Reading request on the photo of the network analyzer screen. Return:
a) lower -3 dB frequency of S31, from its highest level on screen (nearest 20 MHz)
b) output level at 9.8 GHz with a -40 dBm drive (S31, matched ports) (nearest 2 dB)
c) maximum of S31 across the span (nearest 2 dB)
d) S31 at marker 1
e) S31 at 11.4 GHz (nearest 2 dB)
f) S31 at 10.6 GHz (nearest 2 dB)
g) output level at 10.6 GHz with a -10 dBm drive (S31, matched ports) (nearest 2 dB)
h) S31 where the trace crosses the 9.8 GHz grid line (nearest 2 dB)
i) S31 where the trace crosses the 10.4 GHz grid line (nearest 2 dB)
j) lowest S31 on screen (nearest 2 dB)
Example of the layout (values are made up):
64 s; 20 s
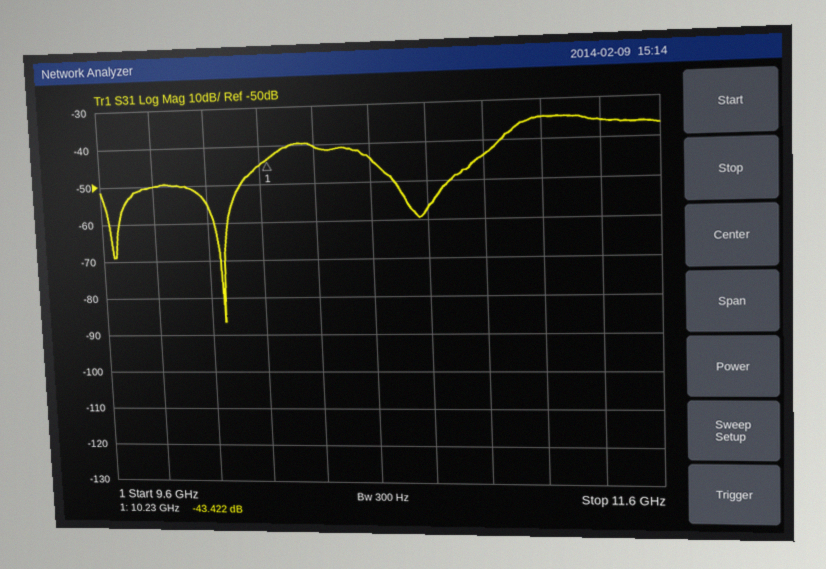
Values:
11.10 GHz; -90 dBm; -34 dB; -43.422 dB; -36 dB; -44 dB; -54 dBm; -50 dB; -40 dB; -86 dB
